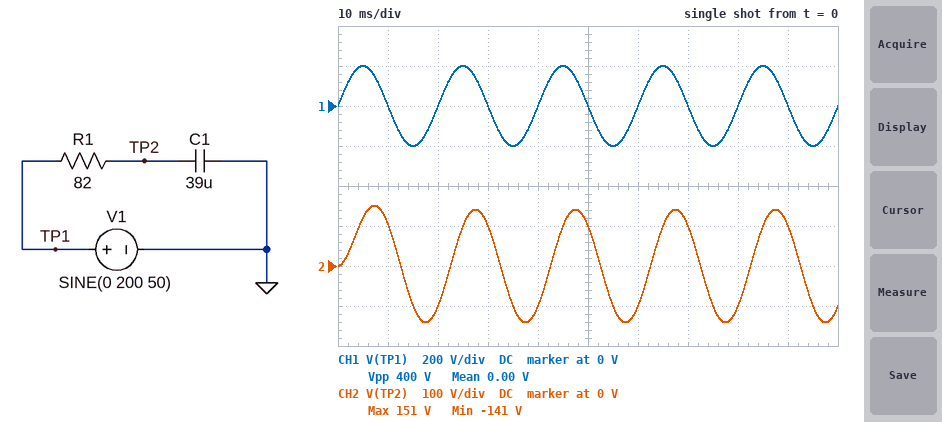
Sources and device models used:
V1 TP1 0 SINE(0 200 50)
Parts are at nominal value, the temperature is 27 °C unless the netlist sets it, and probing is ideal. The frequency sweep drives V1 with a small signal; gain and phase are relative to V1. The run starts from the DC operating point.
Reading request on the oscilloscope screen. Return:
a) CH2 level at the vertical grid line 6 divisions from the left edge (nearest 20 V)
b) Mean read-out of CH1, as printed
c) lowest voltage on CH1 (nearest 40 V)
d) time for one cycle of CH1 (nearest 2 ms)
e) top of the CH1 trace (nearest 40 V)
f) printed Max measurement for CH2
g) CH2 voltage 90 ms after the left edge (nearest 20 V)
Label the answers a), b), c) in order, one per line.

a) -100 V
b) 0.00 V
c) -200 V
d) 20 ms
e) 200 V
f) 151 V
g) 100 V
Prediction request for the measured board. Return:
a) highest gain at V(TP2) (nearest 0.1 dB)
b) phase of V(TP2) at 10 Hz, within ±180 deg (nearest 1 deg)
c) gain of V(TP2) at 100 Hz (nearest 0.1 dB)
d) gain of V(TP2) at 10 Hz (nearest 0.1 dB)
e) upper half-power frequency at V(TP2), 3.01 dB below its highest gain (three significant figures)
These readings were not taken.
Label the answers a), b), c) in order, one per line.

a) 0 dB
b) -11 deg
c) -7.0 dB
d) -0.2 dB
e) 49.8 Hz
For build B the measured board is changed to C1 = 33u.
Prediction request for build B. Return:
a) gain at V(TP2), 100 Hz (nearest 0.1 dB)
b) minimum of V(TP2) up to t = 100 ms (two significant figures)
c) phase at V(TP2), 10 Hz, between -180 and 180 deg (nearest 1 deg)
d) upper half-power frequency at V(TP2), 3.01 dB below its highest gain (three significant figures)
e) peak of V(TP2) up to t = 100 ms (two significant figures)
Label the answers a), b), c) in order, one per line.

a) -5.9 dB
b) -150 V
c) -10 deg
d) 58.8 Hz
e) 160 V
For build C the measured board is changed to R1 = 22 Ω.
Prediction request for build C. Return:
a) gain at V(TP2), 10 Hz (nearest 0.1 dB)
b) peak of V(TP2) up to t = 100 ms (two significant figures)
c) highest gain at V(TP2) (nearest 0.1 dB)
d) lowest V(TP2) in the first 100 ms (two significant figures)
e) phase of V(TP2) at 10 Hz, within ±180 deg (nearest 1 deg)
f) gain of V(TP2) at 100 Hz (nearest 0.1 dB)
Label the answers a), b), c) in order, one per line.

a) 0 dB
b) 190 V
c) 0 dB
d) -190 V
e) -3 deg
f) -1.1 dB
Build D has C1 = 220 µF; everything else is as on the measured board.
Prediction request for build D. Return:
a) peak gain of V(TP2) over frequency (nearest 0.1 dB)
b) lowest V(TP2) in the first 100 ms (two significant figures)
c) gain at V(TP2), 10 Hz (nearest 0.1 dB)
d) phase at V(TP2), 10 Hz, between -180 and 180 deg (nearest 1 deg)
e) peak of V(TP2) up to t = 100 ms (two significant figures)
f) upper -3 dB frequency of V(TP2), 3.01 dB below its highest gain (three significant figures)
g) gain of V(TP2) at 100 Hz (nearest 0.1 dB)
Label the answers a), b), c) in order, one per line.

a) 0 dB
b) -35 V
c) -3.6 dB
d) -49 deg
e) 55 V
f) 8.82 Hz
g) -21.1 dB
